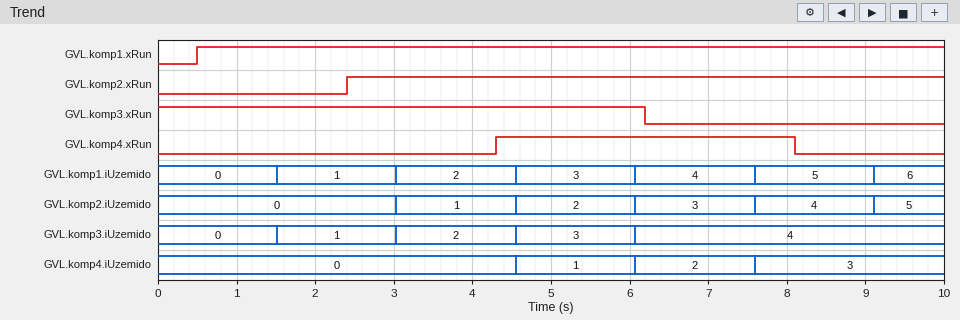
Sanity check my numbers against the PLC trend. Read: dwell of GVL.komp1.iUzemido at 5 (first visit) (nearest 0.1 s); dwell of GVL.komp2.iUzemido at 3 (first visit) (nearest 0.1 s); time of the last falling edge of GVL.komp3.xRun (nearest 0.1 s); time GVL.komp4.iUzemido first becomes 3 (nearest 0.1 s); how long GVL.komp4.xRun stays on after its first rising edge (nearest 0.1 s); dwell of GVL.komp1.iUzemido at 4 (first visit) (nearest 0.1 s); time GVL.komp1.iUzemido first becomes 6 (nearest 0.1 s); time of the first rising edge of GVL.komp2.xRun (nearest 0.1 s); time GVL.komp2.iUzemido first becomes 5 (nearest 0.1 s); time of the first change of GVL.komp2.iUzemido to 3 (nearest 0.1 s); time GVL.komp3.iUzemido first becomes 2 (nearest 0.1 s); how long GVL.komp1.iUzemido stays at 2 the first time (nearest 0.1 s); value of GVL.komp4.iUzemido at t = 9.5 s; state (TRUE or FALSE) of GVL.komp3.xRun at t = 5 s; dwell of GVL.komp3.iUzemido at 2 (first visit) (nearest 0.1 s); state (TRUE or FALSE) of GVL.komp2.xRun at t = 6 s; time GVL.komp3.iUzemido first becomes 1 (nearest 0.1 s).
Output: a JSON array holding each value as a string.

["1.5 s", "1.5 s", "6.2 s", "7.6 s", "3.8 s", "1.5 s", "9.1 s", "2.4 s", "9.1 s", "6.1 s", "3.0 s", "1.5 s", "3", "TRUE", "1.5 s", "TRUE", "1.5 s"]
